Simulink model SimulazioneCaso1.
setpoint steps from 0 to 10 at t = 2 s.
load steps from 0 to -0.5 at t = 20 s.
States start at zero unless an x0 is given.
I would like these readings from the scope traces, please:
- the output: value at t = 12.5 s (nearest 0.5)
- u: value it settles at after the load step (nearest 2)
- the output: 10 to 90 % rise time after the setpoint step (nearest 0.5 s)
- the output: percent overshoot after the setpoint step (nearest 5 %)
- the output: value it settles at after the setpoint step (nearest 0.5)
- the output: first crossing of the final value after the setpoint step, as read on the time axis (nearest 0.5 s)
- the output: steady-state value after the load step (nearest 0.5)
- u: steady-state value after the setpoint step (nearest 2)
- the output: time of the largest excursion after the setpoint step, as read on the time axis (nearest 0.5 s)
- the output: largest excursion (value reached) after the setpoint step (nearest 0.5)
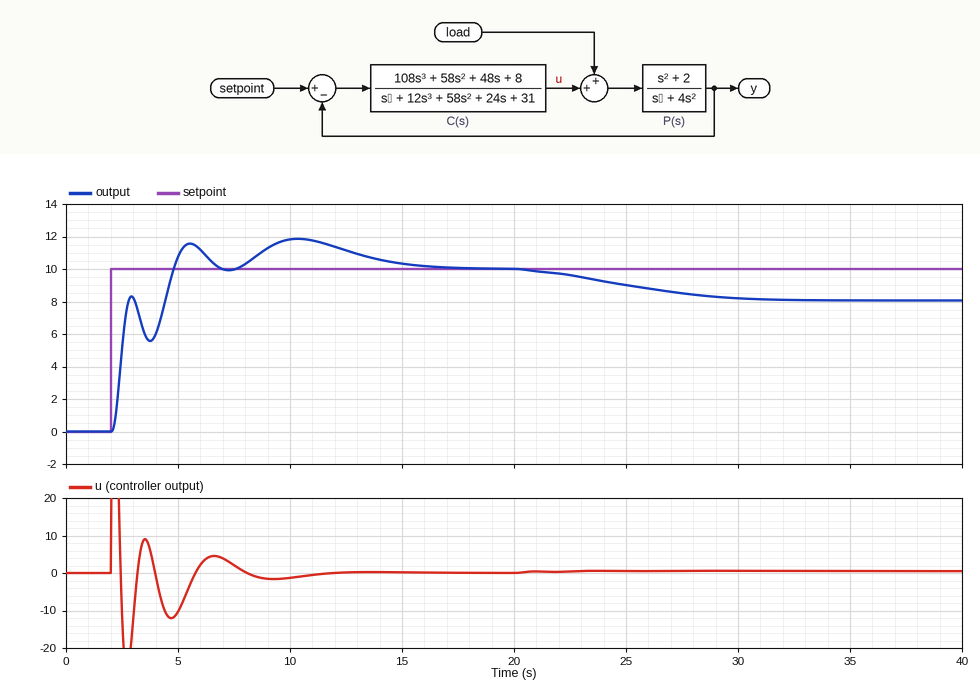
11.0
0
2.5 s
20 %
10.0
5.0 s
8.0
0
10.5 s
12.0
